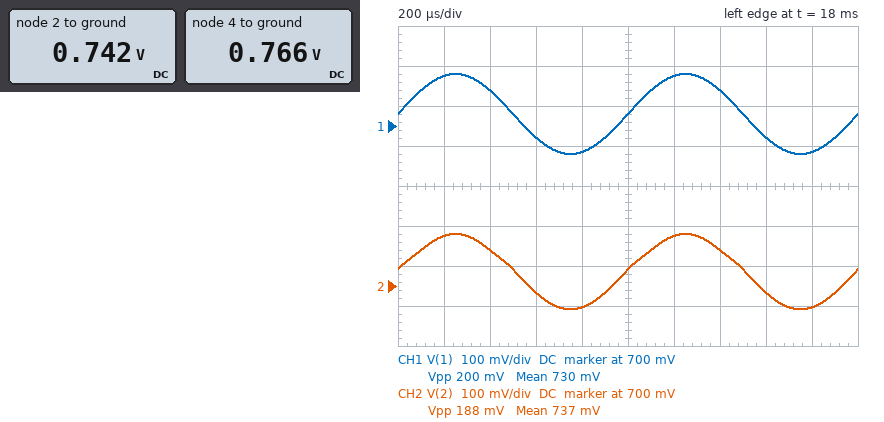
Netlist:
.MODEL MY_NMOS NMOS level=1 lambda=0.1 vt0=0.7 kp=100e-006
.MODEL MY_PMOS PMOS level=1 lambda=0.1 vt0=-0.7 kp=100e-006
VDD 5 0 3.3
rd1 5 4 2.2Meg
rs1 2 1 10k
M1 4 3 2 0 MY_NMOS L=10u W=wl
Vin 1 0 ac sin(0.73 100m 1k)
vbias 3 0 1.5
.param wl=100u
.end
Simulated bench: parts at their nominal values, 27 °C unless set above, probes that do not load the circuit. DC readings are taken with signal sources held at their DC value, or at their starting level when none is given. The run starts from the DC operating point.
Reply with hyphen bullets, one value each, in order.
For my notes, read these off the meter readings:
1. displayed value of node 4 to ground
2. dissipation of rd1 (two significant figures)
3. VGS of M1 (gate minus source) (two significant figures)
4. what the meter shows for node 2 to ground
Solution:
- 0.766 V
- 2.9 µW
- 760 mV
- 0.742 V
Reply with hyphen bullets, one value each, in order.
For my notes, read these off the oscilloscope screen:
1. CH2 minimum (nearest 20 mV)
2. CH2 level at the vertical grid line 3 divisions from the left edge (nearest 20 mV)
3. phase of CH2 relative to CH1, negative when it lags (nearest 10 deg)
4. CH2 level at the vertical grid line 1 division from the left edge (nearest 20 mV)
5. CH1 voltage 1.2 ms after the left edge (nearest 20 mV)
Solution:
- 640 mV
- 680 mV
- 0 deg
- 820 mV
- 820 mV
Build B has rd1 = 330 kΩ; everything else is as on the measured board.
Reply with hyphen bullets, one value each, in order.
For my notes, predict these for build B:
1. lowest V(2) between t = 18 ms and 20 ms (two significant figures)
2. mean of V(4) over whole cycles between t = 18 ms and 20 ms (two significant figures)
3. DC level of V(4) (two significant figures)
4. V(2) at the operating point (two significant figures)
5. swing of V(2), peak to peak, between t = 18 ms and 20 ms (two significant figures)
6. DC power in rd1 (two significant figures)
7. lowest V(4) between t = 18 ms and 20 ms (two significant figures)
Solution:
- 690 mV
- 2.5 V
- 2.7 V
- 750 mV
- 140 mV
- 940 nW
- 1.3 V
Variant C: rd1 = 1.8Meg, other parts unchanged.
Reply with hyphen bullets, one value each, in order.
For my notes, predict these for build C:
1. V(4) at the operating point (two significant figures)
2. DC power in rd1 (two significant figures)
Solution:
- 780 mV
- 3.5 µW
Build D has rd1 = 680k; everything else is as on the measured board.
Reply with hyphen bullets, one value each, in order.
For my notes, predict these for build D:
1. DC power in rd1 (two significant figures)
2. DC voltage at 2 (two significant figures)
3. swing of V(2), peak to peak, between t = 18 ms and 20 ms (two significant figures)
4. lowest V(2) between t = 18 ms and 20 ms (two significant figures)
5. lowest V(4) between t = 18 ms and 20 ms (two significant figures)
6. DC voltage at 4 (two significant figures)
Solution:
- 1.8 µW
- 750 mV
- 160 mV
- 670 mV
- 700 mV
- 2.2 V
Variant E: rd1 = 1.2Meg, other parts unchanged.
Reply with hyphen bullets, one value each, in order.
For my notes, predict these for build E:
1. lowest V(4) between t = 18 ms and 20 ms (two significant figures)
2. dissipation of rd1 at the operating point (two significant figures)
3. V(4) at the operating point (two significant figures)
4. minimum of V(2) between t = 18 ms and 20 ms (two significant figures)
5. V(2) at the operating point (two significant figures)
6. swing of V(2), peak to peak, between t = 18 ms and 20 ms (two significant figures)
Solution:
- 670 mV
- 3.0 µW
- 1.4 V
- 650 mV
- 750 mV
- 180 mV
